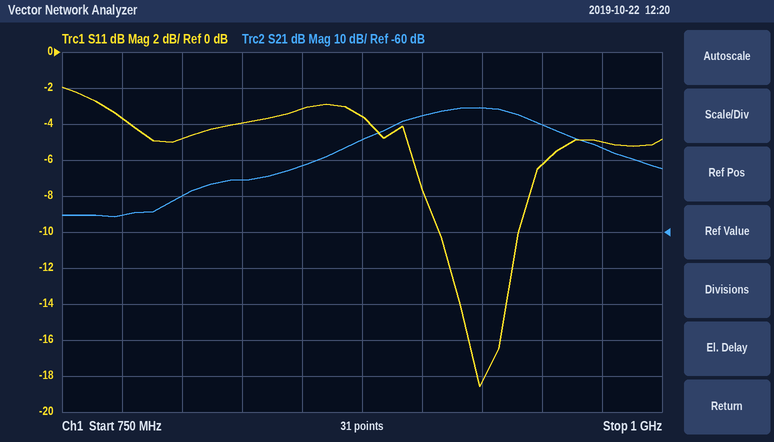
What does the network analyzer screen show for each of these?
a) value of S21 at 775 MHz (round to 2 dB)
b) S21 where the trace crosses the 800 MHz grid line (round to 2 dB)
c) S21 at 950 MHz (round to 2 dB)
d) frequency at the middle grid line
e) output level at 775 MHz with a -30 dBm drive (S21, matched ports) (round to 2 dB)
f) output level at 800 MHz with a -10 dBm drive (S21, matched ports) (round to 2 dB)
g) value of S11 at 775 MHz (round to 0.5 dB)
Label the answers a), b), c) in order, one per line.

a) -56 dB
b) -50 dB
c) -30 dB
d) 875 MHz
e) -86 dBm
f) -60 dBm
g) -3.5 dB
